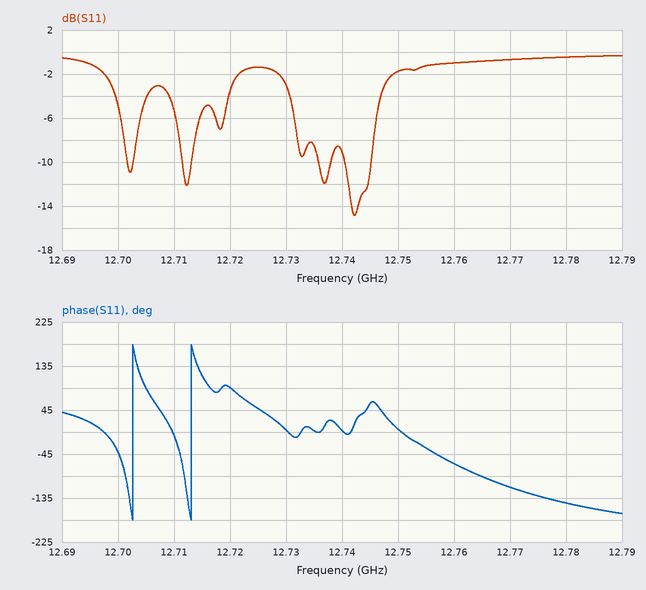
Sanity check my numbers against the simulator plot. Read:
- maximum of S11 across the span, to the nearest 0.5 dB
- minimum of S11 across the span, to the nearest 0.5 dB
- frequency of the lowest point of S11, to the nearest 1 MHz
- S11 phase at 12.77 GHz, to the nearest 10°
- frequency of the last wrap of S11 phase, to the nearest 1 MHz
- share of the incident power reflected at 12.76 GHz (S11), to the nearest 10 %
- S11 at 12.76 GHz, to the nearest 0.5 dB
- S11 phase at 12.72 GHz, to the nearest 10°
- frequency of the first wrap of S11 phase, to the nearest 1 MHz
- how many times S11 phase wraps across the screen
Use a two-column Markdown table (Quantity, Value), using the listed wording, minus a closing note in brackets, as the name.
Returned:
| Quantity | Value |
|---|---|
| maximum of S11 across the span, to the nearest 0.5 dB | -0.5 dB |
| minimum of S11 across the span, to the nearest 0.5 dB | -15.0 dB |
| frequency of the lowest point of S11, to the nearest 1 MHz | 12.742 GHz |
| S11 phase at 12.77 GHz, to the nearest 10° | -110° |
| frequency of the last wrap of S11 phase, to the nearest 1 MHz | 12.713 GHz |
| share of the incident power reflected at 12.76 GHz (S11), to the nearest 10 % | 80 % |
| S11 at 12.76 GHz, to the nearest 0.5 dB | -1.0 dB |
| S11 phase at 12.72 GHz, to the nearest 10° | 90° |
| frequency of the first wrap of S11 phase, to the nearest 1 MHz | 12.703 GHz |
| how many times S11 phase wraps across the screen | 2 |
